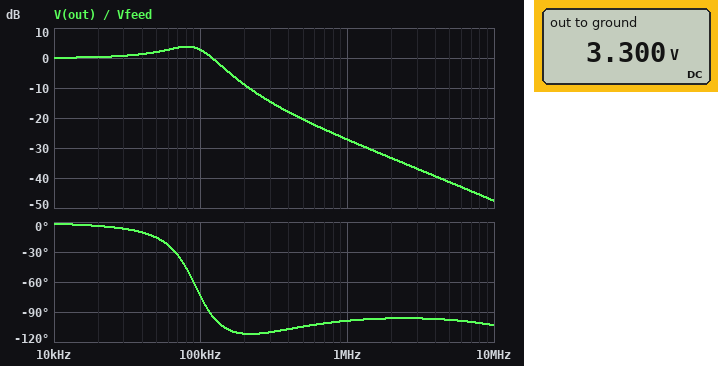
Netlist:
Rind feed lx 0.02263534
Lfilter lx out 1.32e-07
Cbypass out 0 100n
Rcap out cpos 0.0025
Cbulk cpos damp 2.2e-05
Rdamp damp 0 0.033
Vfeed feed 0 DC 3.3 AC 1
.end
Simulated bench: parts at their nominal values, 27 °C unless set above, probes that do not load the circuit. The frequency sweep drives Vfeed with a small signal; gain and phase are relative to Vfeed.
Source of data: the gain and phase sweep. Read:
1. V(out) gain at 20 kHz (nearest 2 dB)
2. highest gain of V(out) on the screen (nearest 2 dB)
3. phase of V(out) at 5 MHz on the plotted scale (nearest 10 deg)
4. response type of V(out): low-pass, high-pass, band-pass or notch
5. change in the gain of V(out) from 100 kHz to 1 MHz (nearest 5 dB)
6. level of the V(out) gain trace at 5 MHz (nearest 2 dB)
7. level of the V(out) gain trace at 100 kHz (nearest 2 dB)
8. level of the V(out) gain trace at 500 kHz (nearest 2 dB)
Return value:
0 dB
4 dB
-100 deg
low-pass
-30 dB
-42 dB
2 dB
-20 dB
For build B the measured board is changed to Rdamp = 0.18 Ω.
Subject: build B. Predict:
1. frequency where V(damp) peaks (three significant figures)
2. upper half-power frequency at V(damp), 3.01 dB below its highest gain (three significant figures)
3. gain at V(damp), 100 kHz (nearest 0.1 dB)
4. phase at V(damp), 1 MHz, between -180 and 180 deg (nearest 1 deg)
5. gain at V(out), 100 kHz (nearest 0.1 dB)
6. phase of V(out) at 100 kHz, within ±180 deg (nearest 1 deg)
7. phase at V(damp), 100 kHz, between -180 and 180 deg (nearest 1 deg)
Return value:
94.4 kHz
283 kHz
-1.1 dB
-82 deg
-0.4 dB
-25 deg
-3 deg
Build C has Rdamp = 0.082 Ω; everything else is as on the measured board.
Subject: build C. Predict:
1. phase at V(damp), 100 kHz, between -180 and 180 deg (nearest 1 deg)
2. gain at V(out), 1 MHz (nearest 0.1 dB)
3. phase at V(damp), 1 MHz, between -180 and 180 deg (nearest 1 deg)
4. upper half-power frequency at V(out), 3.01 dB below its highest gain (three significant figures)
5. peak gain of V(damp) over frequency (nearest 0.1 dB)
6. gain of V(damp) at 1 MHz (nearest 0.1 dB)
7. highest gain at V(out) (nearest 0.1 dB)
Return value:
-6 deg
-19.8 dB
-86 deg
136 kHz
-2.3 dB
-20.1 dB
1.2 dB
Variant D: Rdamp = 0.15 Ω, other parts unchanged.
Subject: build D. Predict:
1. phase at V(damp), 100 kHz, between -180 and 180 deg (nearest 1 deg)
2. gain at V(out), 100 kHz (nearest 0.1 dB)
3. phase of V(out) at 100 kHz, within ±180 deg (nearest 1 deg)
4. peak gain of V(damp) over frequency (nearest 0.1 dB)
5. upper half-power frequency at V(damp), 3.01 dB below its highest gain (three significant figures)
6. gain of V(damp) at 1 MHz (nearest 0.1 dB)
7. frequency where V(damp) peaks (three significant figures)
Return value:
-4 deg
-0.3 dB
-29 deg
-1.3 dB
249 kHz
-14.9 dB
94.0 kHz
